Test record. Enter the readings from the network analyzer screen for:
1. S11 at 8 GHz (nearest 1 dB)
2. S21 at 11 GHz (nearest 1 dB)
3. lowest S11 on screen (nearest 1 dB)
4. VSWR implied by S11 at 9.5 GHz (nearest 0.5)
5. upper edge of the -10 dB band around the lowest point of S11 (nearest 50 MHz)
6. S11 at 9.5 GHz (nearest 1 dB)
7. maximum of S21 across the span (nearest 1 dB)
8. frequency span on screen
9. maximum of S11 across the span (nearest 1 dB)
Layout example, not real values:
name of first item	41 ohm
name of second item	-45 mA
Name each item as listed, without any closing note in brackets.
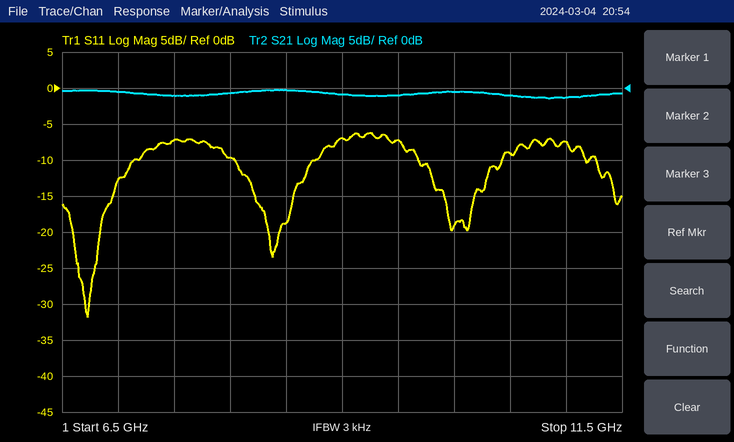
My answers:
S11 at 8 GHz	-10 dB
S21 at 11 GHz	-1 dB
lowest S11 on screen	-32 dB
VSWR implied by S11 at 9.5 GHz	2.5
upper edge of the -10 dB band around the lowest point of S11	7.15 GHz
S11 at 9.5 GHz	-7 dB
maximum of S21 across the span	0 dB
frequency span on screen	5 GHz
maximum of S11 across the span	-6 dB
